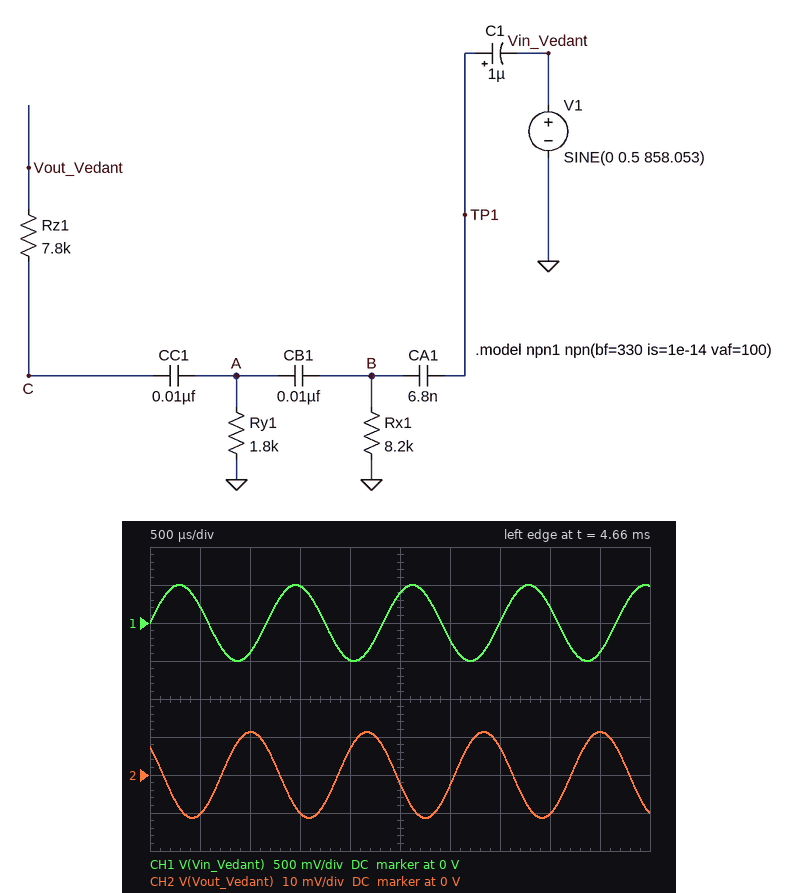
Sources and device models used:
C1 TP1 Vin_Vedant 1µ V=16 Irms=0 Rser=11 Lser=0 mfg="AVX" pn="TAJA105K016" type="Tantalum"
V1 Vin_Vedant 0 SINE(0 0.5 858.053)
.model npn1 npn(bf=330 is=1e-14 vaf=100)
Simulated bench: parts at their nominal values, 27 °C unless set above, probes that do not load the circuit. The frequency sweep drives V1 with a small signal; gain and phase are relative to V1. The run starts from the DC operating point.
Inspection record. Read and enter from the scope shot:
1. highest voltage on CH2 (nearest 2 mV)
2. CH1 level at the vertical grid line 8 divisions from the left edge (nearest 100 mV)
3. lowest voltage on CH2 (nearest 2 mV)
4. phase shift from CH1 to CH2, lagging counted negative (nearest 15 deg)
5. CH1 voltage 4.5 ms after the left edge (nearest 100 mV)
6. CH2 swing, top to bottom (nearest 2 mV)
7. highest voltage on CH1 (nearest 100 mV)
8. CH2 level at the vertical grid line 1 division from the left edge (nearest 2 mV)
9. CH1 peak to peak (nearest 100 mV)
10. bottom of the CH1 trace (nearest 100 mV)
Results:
12 mV
200 mV
-12 mV
135 deg
-400 mV
22 mV
500 mV
-10 mV
1.0 V
-500 mV
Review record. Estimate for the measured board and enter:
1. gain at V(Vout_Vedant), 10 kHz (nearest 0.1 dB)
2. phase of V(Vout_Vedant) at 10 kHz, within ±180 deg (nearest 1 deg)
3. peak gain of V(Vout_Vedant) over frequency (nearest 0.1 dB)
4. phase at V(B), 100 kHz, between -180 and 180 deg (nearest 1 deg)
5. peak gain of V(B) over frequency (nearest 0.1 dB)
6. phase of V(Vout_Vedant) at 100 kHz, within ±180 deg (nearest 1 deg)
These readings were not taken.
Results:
-8.3 dB
73 deg
-0.1 dB
9 deg
-0.1 dB
14 deg
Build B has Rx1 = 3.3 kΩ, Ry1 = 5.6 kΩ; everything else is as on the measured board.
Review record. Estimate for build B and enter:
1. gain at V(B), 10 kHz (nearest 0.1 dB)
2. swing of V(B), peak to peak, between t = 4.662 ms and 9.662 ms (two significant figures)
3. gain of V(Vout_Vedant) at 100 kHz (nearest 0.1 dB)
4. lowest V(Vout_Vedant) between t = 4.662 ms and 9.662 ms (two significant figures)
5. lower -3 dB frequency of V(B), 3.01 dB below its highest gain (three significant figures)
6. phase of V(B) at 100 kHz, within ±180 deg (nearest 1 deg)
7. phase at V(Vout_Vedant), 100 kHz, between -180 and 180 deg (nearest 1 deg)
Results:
-3.9 dB
110 mV
-0.1 dB
-16 mV
12.1 kHz
6 deg
8 deg
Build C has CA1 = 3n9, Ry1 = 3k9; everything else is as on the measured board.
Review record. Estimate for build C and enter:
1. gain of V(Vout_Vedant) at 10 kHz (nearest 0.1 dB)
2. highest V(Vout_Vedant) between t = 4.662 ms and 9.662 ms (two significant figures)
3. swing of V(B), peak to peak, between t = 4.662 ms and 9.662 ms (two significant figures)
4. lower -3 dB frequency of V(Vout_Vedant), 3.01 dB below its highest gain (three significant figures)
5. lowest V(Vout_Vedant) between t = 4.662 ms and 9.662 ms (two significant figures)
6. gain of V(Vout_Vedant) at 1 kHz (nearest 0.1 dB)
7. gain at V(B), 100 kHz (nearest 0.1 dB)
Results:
-6.5 dB
14 mV
140 mV
18.5 kHz
-14 mV
-28.8 dB
-0.2 dB
